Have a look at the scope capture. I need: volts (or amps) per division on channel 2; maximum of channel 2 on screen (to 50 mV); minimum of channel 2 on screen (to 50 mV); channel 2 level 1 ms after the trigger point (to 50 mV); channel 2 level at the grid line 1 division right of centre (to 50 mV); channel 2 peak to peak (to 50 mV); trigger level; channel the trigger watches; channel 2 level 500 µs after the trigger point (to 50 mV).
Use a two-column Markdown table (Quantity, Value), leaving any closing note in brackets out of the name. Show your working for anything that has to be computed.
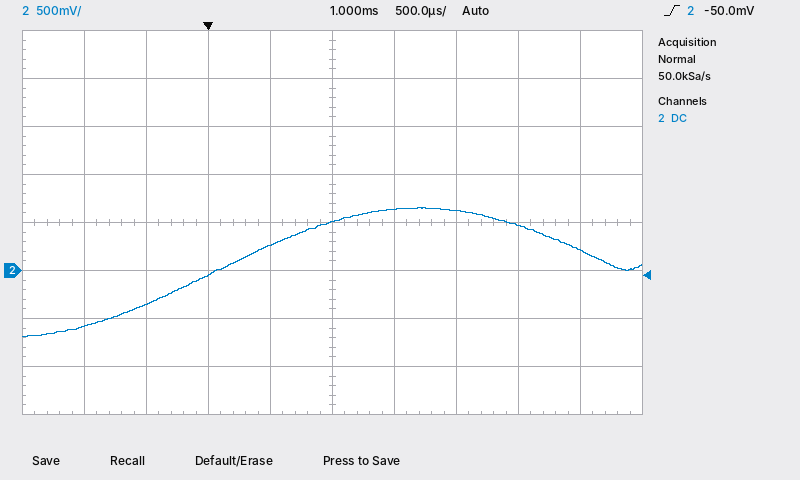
| Quantity | Value |
|---|---|
| volts (or amps) per division on channel 2 | 500 mV |
| maximum of channel 2 on screen | 650 mV |
| minimum of channel 2 on screen | -700 mV |
| channel 2 level 1 ms after the trigger point | 500 mV |
| channel 2 level at the grid line 1 division right of centre | 650 mV |
| channel 2 peak to peak | 650 mV − (-700 mV) = 1.35 V |
| trigger level | -50.0 mV |
| channel the trigger watches | channel 2 |
| channel 2 level 500 µs after the trigger point | 250 mV |
